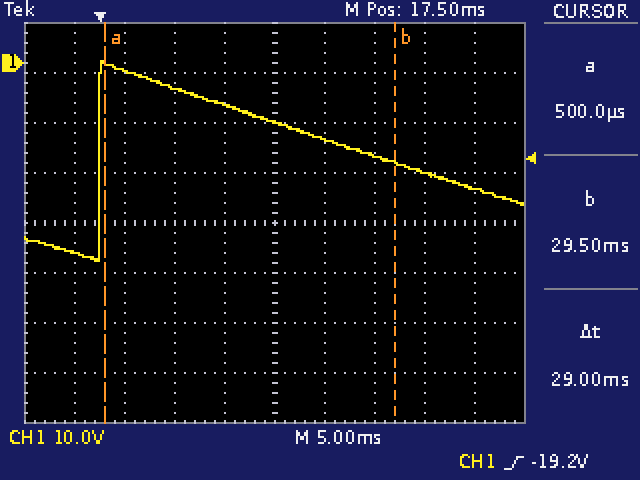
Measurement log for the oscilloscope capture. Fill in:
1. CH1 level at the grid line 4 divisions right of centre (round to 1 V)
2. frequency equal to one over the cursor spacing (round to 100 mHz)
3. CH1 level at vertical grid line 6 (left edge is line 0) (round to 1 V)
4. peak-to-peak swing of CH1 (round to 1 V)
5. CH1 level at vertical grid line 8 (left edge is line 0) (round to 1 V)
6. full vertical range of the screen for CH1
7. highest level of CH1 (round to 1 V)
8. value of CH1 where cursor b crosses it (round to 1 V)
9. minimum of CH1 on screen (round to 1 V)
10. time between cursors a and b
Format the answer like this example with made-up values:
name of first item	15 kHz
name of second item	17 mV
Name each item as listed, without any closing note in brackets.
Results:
CH1 level at the grid line 4 divisions right of centre	-25 V
frequency equal to one over the cursor spacing	34.5 Hz
CH1 level at vertical grid line 6 (left edge is line 0)	-15 V
peak-to-peak swing of CH1	40 V
CH1 level at vertical grid line 8 (left edge is line 0)	-22 V
full vertical range of the screen for CH1	80 V
highest level of CH1	0 V
value of CH1 where cursor b crosses it	-20 V
minimum of CH1 on screen	-40 V
time between cursors a and b	29 ms
